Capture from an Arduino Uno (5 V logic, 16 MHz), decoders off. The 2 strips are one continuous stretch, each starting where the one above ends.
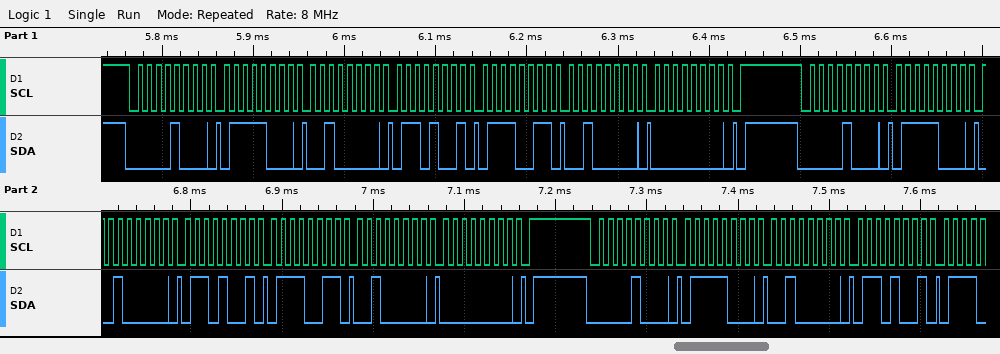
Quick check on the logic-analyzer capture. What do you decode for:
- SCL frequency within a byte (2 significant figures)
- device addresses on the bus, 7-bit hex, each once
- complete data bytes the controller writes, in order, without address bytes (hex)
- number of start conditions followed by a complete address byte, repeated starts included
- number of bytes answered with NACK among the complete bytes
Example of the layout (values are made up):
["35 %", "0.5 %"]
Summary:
["100 kHz", "0x04", "78 20 69 73 20 00 78 20 69 73 20 00 78 20 69", "3", "0"]
